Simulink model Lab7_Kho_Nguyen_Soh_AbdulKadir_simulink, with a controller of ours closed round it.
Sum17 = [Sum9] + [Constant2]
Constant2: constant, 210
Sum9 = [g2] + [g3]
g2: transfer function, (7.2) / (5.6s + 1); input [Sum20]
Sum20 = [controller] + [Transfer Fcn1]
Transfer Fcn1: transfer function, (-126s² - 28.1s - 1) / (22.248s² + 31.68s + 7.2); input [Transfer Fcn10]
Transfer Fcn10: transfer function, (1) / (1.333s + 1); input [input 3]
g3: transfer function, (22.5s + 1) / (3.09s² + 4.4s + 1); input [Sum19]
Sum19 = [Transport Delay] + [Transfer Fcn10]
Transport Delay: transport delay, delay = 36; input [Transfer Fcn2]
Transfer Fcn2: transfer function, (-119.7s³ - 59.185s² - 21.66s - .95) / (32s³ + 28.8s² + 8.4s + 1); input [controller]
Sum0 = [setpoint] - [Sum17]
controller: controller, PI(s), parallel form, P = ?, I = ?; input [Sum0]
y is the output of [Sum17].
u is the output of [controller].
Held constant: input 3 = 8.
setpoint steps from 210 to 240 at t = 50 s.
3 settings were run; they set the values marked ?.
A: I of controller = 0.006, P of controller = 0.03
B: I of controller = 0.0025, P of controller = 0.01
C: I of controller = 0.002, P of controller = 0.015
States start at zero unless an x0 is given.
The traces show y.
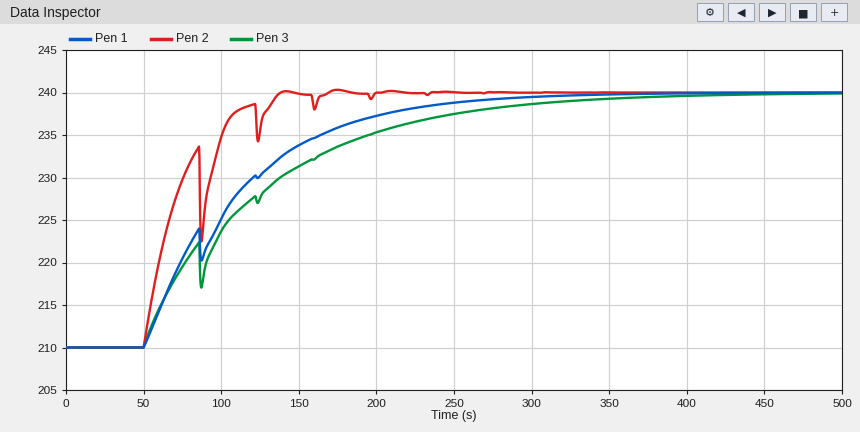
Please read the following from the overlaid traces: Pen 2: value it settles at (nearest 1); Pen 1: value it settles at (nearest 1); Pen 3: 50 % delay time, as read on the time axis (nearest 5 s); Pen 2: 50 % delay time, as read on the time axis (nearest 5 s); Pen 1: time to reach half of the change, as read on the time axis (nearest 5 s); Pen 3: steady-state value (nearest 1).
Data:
240
240
105 s
65 s
100 s
240
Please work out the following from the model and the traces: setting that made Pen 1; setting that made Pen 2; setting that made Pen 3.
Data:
B
A
C
